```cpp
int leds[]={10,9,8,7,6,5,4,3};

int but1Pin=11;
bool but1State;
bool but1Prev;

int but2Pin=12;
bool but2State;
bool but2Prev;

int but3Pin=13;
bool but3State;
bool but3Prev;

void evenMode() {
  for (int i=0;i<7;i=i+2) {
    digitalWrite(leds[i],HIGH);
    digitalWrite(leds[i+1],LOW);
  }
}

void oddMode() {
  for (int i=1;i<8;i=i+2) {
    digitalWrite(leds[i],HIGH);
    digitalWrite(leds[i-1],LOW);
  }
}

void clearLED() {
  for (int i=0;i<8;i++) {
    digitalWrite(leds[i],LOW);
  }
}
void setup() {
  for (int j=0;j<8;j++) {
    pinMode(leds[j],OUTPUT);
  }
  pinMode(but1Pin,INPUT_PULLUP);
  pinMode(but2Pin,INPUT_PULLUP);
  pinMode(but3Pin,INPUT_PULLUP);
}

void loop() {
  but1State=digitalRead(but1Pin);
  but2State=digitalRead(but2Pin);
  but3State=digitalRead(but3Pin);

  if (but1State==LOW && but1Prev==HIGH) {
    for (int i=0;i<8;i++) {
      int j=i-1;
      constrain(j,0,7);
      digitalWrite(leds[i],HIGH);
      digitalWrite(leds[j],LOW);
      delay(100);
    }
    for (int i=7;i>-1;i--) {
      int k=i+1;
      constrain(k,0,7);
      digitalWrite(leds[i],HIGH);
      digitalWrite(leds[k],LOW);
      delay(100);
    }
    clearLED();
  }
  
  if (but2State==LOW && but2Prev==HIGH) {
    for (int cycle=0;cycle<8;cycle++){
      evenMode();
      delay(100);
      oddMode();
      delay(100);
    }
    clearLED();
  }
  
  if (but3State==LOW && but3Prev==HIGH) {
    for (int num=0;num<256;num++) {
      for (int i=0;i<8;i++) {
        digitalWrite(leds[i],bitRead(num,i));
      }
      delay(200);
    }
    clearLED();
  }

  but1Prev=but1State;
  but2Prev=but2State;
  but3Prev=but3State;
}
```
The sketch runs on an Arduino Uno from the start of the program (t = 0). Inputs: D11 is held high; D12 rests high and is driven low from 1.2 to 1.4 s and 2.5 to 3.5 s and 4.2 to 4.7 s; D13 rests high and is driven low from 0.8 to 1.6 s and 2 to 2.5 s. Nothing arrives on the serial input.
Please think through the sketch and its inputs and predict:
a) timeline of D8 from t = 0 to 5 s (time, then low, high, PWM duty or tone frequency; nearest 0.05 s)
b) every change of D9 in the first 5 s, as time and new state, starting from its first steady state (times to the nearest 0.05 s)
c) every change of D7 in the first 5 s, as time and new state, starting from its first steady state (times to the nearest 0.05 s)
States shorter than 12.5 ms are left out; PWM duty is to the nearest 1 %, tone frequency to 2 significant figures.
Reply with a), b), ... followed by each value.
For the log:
a) 0 s low; 1.6 s high; 2.4 s low; 3.2 s high; 4 s low; 4.8 s high
b) 0 s low; 1.2 s high; 1.6 s low; 2 s high; 2.4 s low; 2.8 s high; 3.2 s low; 3.6 s high; 4 s low; 4.4 s high; 4.8 s low
c) 0 s low; 2.4 s high; 4 s low
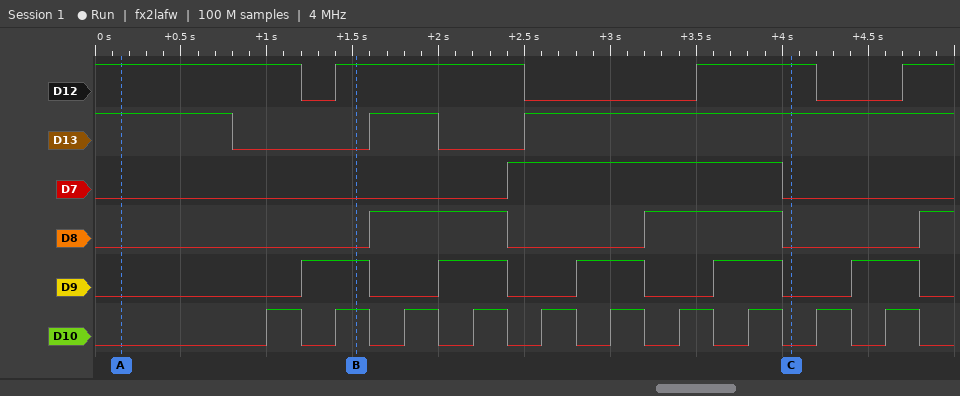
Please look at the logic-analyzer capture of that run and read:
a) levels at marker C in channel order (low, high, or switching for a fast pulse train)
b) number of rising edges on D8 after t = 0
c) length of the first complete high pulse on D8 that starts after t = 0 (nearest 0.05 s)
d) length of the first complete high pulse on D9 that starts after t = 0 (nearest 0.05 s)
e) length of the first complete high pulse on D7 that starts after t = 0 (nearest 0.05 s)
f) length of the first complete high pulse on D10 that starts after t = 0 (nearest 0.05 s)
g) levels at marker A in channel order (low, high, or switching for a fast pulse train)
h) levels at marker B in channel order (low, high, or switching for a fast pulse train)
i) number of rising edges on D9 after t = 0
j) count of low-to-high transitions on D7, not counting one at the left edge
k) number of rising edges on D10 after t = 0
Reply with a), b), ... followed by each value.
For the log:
a) D12 high, D13 high, D7 low, D8 low, D9 low, D10 low
b) 3
c) 0.80 s
d) 0.40 s
e) 1.60 s
f) 0.20 s
g) D12 high, D13 high, D7 low, D8 low, D9 low, D10 low
h) D12 high, D13 low, D7 low, D8 low, D9 high, D10 high
i) 5
j) 1
k) 10
